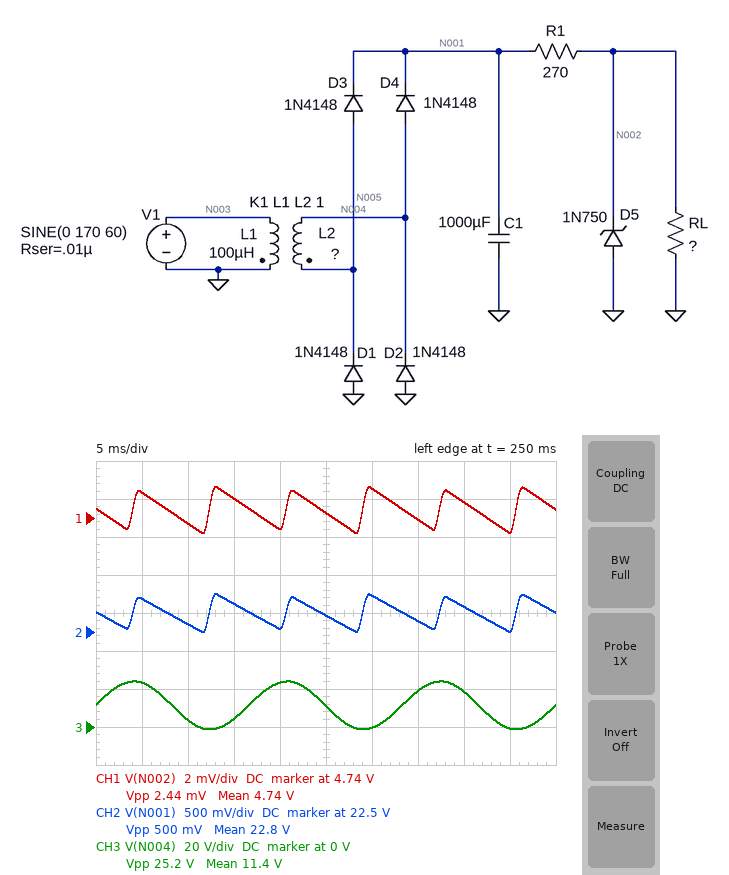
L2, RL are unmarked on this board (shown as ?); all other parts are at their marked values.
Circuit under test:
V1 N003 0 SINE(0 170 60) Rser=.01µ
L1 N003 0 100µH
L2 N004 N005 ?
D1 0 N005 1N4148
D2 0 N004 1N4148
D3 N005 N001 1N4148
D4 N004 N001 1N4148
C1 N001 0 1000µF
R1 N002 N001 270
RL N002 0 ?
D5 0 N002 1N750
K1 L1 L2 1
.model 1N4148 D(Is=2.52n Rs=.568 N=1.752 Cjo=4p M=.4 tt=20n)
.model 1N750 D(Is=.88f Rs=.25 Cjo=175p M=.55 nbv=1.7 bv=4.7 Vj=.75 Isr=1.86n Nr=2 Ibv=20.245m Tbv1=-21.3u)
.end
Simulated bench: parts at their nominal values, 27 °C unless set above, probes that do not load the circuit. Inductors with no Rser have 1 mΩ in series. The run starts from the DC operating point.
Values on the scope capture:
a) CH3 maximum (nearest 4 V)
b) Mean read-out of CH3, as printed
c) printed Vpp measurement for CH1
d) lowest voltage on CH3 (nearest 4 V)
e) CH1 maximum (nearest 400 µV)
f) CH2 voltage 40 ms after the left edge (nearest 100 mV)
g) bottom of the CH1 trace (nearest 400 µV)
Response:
24 V
11.4 V
2.44 mV
0 V
4.7416 V
22.8 V
4.7392 V
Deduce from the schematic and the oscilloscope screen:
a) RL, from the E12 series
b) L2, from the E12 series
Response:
180 Ω
2.2 µH
